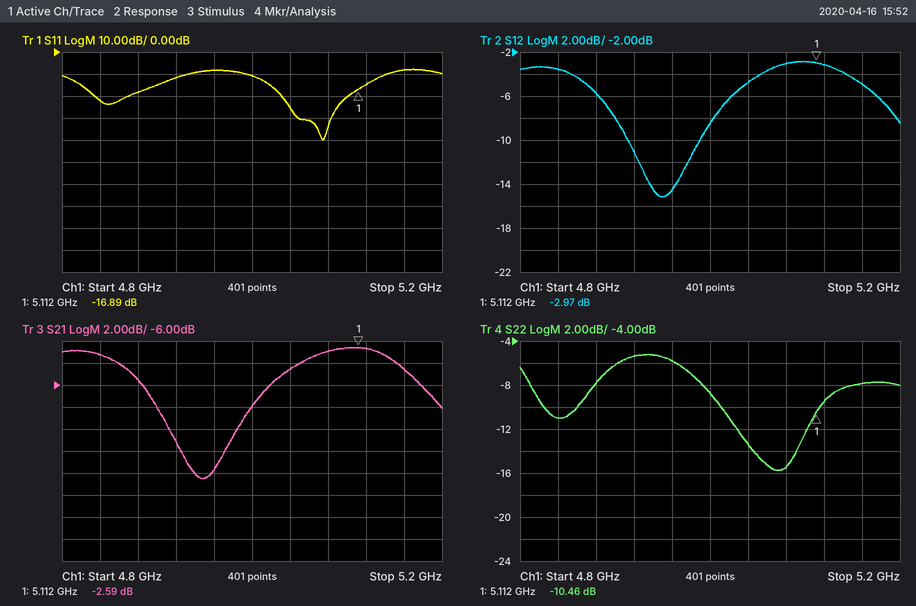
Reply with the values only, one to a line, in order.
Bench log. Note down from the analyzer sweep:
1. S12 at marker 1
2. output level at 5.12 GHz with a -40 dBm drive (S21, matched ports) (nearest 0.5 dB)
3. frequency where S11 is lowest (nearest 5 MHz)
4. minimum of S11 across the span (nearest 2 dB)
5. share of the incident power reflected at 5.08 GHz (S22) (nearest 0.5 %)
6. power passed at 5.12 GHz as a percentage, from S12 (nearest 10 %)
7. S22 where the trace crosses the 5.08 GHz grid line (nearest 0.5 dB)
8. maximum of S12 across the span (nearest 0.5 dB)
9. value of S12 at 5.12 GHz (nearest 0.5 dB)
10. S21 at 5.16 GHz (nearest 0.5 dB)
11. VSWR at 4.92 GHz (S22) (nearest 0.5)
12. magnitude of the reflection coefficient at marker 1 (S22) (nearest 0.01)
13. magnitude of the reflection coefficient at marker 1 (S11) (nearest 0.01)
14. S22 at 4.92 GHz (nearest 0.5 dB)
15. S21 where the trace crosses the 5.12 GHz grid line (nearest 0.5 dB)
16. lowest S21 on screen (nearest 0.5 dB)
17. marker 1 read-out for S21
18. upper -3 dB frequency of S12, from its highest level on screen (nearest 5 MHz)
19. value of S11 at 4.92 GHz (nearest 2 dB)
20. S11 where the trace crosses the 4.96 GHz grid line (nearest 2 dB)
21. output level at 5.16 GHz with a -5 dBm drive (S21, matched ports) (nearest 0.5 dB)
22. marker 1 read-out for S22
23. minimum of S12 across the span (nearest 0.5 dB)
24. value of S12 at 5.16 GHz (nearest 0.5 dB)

-2.97 dB
-42.5 dBm
5.075 GHz
-40 dB
3.0 %
50 %
-15.5 dB
-3.0 dB
-3.0 dB
-4.5 dB
3.5
0.30
0.14
-5.5 dB
-2.5 dB
-14.5 dB
-2.59 dB
5.175 GHz
-12 dB
-8 dB
-9.5 dBm
-10.46 dB
-15.0 dB
-5.0 dB
